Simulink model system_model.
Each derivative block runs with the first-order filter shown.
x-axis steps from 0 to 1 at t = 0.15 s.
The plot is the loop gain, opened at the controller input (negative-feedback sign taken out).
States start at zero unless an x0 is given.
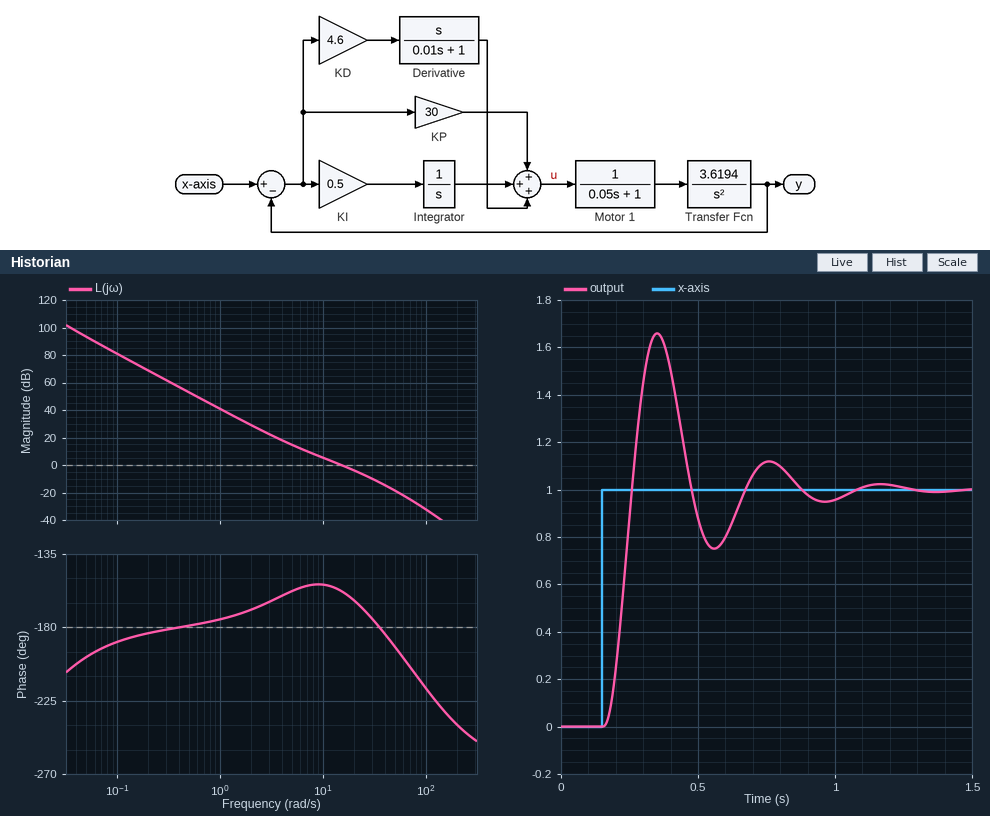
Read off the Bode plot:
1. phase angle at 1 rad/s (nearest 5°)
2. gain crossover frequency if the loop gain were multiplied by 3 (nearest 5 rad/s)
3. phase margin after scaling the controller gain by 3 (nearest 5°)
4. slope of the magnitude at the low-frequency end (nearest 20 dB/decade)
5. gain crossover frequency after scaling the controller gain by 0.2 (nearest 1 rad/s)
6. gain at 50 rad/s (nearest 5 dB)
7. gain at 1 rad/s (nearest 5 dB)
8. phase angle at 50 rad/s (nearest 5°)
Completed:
-175°
30 rad/s
5°
-40 dB/decade
5 rad/s
-20 dB
40 dB
-190°
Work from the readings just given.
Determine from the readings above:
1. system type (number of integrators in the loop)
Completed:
2
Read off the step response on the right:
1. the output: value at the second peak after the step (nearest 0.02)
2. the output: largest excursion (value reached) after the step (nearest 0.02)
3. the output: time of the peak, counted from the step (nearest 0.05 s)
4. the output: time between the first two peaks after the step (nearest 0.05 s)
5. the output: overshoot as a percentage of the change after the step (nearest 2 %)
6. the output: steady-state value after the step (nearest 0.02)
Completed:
1.12
1.66
0.20 s
0.40 s
66 %
1.00
